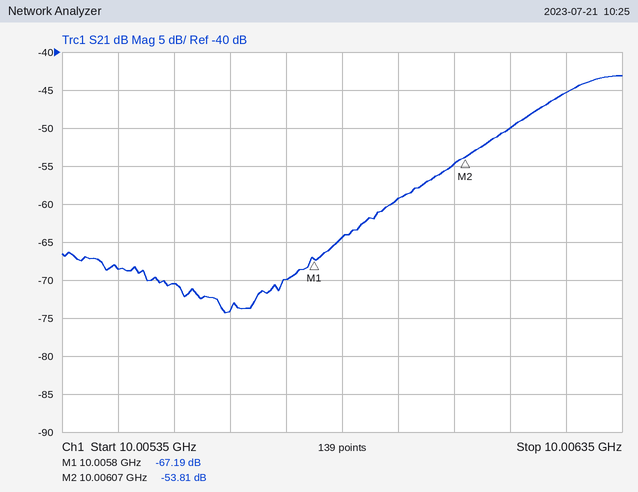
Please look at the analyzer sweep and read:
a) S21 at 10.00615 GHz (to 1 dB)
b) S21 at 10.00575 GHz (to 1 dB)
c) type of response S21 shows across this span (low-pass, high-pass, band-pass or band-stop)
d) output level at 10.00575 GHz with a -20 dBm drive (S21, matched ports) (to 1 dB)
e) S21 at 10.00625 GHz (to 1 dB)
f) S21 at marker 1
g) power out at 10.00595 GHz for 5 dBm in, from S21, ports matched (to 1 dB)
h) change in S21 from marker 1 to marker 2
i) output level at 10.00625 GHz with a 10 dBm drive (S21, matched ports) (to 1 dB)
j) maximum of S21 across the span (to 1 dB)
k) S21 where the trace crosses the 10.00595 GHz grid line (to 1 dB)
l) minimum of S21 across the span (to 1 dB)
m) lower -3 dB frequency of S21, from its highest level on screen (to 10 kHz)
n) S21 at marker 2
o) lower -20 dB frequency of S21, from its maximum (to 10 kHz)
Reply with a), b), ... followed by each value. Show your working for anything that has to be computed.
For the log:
a) -50 dB
b) -70 dB
c) high-pass
d) -20 dBm + (-70 dB) = -90 dBm
e) -45 dB
f) -67.19 dB
g) 5 dBm + (-59 dB) = -54 dBm
h) -53.81 − (-67.19) = 13.38 dB
i) 10 dBm + (-45 dB) = -35 dBm
j) -43 dB
k) -59 dB
l) -74 dB
m) 10.00623 GHz
n) -53.81 dB
o) 10.00588 GHz
